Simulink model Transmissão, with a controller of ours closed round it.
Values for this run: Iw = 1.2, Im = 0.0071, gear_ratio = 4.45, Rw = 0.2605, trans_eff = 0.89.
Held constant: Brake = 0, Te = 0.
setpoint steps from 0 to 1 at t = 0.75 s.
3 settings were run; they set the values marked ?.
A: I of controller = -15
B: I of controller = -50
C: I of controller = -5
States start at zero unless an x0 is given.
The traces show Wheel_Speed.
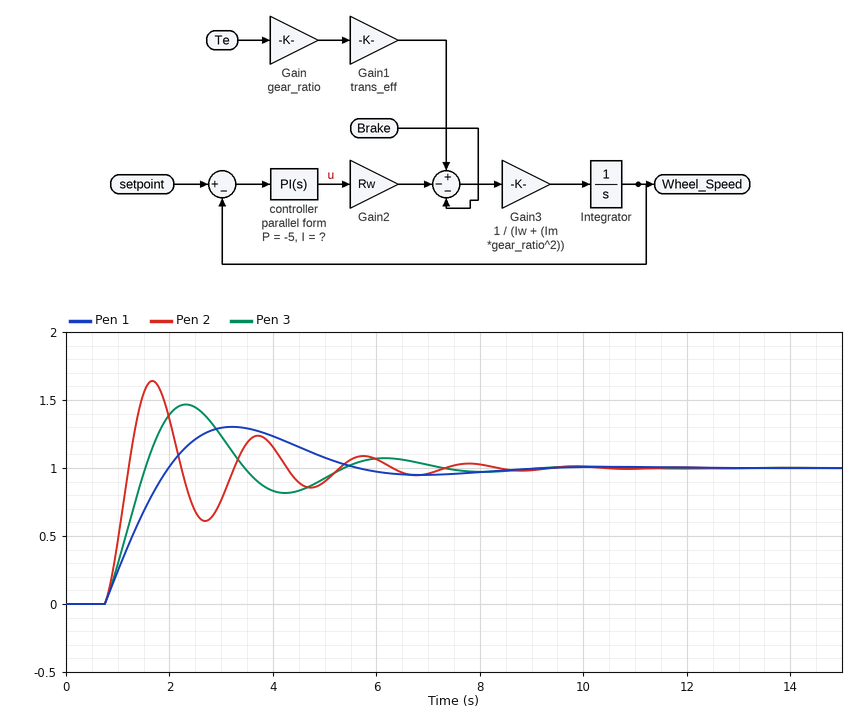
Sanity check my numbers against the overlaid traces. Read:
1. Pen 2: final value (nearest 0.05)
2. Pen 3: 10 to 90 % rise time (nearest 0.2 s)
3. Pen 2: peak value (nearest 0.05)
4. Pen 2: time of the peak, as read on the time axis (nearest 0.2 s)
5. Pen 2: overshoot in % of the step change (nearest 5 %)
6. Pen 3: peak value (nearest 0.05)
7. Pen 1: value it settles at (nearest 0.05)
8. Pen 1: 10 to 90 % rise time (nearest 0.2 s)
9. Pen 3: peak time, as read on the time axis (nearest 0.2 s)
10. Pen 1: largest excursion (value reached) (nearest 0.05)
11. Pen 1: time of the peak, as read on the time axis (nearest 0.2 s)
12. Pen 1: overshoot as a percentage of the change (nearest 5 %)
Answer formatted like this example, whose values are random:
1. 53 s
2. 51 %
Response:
1. 1.00
2. 0.6 s
3. 1.65
4. 1.6 s
5. 65 %
6. 1.45
7. 1.00
8. 1.0 s
9. 2.4 s
10. 1.30
11. 3.2 s
12. 30 %
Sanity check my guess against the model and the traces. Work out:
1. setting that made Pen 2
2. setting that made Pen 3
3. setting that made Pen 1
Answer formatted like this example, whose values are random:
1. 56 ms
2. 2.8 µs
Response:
1. B
2. A
3. C
